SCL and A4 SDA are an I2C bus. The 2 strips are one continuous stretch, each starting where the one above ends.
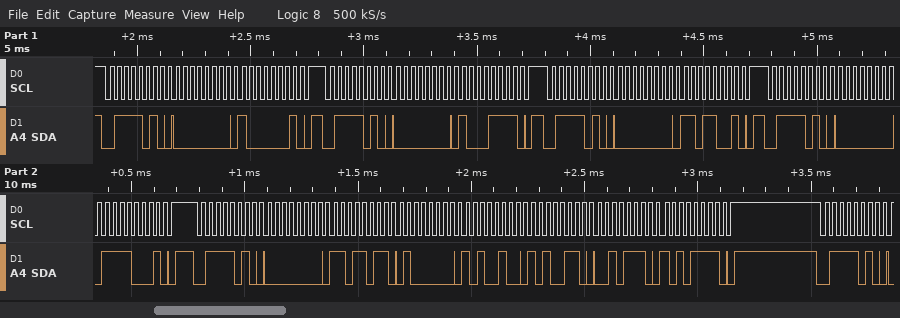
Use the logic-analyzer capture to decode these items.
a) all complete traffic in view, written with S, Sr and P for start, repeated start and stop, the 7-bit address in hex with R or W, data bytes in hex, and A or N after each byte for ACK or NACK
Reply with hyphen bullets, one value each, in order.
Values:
- S 3DW A 00 A 81 A P S 3DW A 00 A 8F A P S 3DW A 00 A D9 A P S 3DW A 00 A F1 A P S 3DW A 00 A DB A 40 A A4 A A6 A 2E A AF A P S 3DW A
